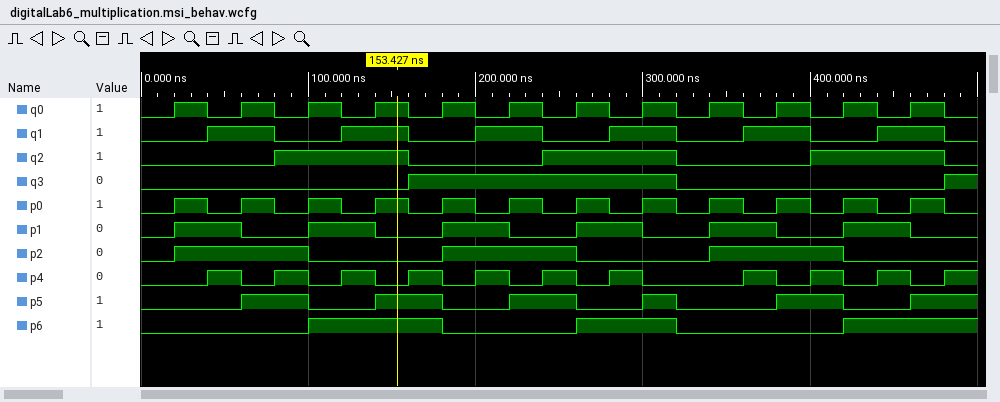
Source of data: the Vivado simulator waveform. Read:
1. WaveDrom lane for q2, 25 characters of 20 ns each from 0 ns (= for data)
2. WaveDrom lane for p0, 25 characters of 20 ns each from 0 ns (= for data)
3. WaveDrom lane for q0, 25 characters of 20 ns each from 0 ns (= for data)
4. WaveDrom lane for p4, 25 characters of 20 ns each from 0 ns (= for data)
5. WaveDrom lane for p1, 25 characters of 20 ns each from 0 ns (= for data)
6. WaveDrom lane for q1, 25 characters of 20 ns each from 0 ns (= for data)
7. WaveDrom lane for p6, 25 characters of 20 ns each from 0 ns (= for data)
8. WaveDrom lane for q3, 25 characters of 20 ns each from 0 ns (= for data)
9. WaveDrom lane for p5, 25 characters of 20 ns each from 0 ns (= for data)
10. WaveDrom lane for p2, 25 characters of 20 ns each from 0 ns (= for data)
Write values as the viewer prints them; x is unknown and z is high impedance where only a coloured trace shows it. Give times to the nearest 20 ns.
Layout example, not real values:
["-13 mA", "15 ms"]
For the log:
["{name: 'q2', wave: '0...1...0...1...0...1...0'}", "{name: 'p0', wave: '0101010101010101010101010'}", "{name: 'q0', wave: '0101010101010101010101010'}", "{name: 'p4', wave: '0.10101010101010..1010101'}", "{name: 'p1', wave: '01.0.1.0.1.0.1.0.1.0.1.0.'}", "{name: 'q1', wave: '0.1.0.1.0.1.0.1.0.1.0.1.0'}", "{name: 'p6', wave: '0....1...0...1..0....1...'}", "{name: 'q3', wave: '0.......1.......0.......1'}", "{name: 'p5', wave: '0..1.0.1.0.1.0.10..1.0.1.'}", "{name: 'p2', wave: '01...0...1...0...1...0...'}"]
